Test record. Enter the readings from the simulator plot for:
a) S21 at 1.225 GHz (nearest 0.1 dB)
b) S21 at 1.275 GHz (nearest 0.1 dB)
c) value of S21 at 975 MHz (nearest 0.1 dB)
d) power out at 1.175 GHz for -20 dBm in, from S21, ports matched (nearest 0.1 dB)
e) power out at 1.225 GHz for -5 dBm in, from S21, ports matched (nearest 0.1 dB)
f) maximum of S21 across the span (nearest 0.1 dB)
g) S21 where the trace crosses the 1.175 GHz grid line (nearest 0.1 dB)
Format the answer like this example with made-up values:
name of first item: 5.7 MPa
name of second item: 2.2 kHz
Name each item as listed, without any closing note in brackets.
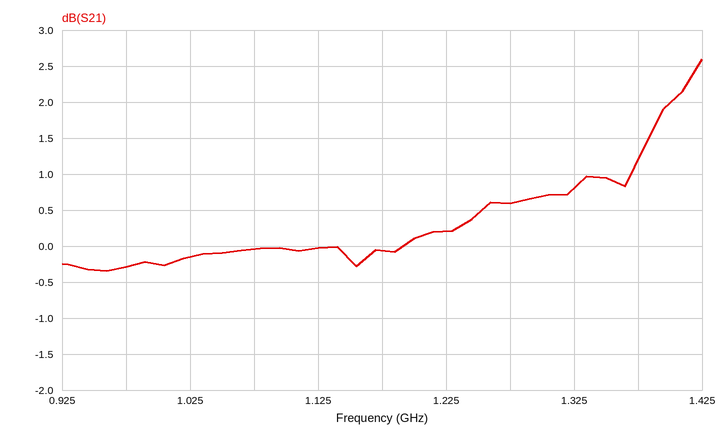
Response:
S21 at 1.225 GHz: 0.2 dB
S21 at 1.275 GHz: 0.6 dB
value of S21 at 975 MHz: -0.3 dB
power out at 1.175 GHz for -20 dBm in, from S21, ports matched: -20.1 dBm
power out at 1.225 GHz for -5 dBm in, from S21, ports matched: -4.8 dBm
maximum of S21 across the span: 2.6 dB
S21 where the trace crosses the 1.175 GHz grid line: -0.1 dB
